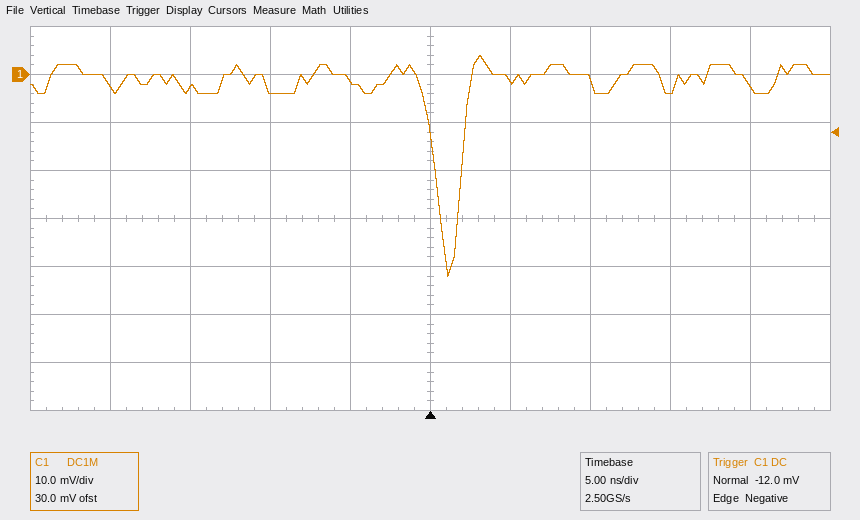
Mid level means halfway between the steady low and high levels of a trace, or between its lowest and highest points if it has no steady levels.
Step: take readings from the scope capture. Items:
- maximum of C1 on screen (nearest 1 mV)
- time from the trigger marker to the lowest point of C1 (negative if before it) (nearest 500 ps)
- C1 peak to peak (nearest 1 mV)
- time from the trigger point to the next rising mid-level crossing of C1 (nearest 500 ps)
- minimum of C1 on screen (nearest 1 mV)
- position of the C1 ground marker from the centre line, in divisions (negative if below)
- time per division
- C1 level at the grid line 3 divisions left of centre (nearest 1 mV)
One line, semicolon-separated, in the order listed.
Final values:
4 mV; +1.0 ns; 46 mV; 2.0 ns; -42 mV; +3.0 div; 5 ns; -3 mV
